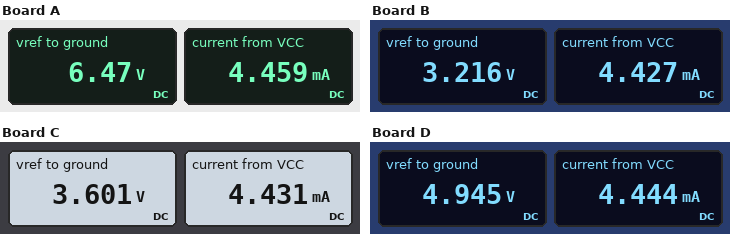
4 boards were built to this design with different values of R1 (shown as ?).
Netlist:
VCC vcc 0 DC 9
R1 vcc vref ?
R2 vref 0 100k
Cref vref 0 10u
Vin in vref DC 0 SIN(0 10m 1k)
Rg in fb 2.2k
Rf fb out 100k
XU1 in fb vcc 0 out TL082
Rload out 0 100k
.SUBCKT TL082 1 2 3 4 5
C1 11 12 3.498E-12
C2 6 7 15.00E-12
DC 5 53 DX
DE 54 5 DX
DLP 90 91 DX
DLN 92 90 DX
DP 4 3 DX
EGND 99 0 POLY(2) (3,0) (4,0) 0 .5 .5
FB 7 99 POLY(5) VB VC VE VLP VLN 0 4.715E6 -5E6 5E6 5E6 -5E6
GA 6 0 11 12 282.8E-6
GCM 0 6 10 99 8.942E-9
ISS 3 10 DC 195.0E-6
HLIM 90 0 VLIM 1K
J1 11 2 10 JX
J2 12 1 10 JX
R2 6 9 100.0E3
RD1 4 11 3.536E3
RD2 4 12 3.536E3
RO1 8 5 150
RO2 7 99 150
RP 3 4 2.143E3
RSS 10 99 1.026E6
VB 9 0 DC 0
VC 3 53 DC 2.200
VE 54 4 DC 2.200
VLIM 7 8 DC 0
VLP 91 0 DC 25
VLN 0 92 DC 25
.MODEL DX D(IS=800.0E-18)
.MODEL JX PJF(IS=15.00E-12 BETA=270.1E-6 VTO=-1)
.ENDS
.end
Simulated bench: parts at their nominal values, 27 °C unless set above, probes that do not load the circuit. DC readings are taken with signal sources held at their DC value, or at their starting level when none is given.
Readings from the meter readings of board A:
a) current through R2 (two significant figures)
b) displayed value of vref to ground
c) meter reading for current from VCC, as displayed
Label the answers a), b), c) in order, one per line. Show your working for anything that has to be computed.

a) (6.47 V) / 100 kΩ = 65 µA
b) 6.47 V
c) 4.459 mA
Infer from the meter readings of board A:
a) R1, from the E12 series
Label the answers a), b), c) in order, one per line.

a) 39 kΩ
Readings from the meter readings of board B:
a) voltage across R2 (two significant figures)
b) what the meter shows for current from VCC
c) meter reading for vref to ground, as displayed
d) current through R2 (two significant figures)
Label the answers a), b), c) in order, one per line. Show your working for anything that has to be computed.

a) 3.216 V = 3.2 V
b) 4.427 mA
c) 3.216 V
d) (3.216 V) / 100 kΩ = 32 µA
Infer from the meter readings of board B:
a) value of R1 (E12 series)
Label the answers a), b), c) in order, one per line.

a) 180 kΩ
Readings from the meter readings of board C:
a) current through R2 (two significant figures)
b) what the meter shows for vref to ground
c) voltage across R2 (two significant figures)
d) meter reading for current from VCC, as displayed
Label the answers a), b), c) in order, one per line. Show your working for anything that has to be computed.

a) (3.601 V) / 100 kΩ = 36 µA
b) 3.601 V
c) 3.601 V = 3.6 V
d) 4.431 mA
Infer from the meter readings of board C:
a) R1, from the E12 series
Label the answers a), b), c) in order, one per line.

a) 150 kΩ
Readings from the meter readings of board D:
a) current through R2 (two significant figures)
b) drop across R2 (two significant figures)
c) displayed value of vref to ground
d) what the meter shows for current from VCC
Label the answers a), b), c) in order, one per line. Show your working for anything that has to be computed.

a) (4.945 V) / 100 kΩ = 49 µA
b) 4.945 V = 4.9 V
c) 4.945 V
d) 4.444 mA
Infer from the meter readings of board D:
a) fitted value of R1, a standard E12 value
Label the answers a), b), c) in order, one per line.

a) 82 kΩ
